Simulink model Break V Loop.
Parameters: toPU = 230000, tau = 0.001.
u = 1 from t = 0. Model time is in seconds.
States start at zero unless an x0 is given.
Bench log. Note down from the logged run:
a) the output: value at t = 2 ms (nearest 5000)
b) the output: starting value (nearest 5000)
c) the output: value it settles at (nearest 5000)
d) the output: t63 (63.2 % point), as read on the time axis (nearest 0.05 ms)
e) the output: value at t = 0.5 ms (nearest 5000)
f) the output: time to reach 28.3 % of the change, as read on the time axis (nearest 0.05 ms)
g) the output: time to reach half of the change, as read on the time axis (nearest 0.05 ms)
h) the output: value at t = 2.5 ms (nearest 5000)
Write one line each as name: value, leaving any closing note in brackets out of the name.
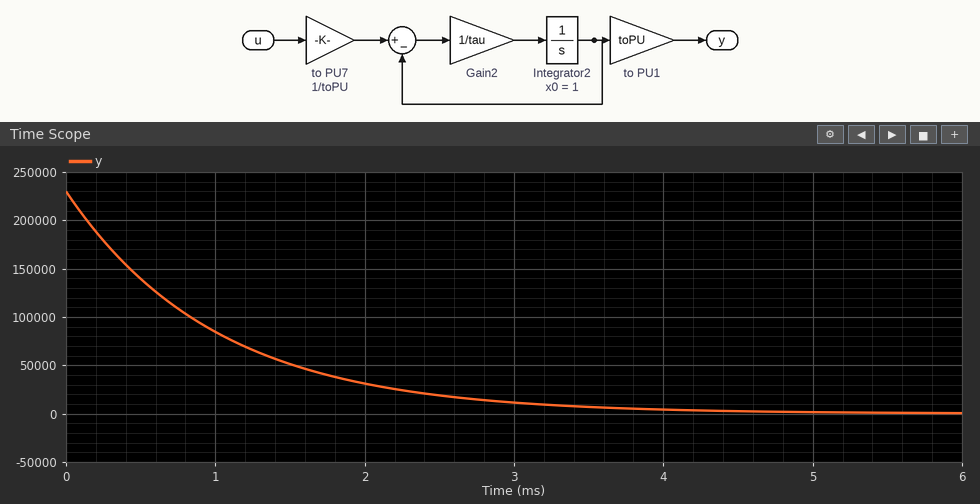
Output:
the output: value at t = 2 ms: 30000
the output: starting value: 230000
the output: value it settles at: 0
the output: t63 (63.2 % point), as read on the time axis: 1.00 ms
the output: value at t = 0.5 ms: 140000
the output: time to reach 28.3 % of the change, as read on the time axis: 0.35 ms
the output: time to reach half of the change, as read on the time axis: 0.70 ms
the output: value at t = 2.5 ms: 20000
